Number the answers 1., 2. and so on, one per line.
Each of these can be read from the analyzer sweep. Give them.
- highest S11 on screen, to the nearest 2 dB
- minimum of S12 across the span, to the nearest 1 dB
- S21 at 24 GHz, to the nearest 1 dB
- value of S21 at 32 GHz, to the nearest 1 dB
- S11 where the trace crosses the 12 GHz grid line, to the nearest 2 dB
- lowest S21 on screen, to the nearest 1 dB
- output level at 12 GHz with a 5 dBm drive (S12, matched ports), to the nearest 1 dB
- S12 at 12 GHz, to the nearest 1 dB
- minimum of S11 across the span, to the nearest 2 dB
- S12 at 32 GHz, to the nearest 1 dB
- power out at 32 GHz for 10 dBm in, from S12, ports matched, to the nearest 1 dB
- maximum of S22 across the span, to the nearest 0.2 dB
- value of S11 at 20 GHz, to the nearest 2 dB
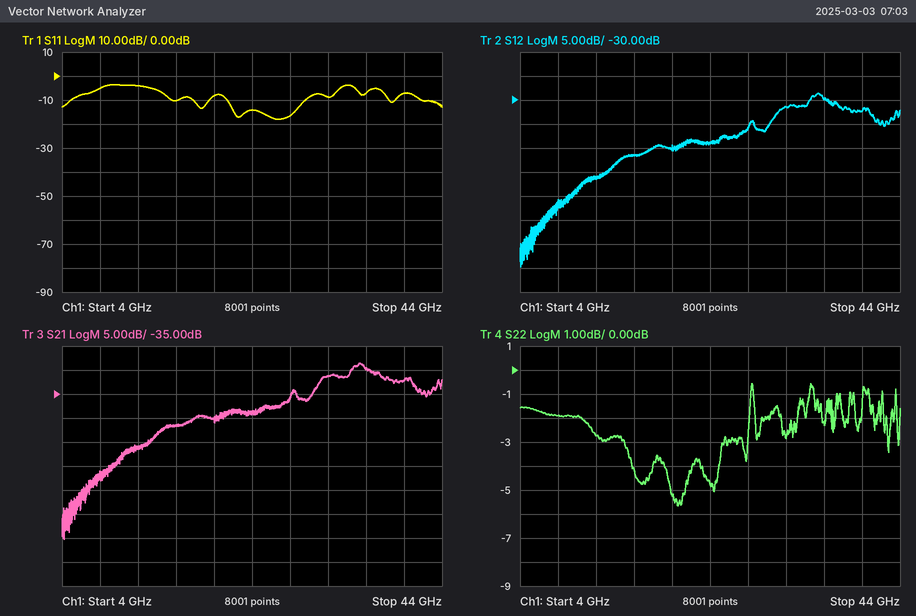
1. -4 dB
2. -65 dB
3. -39 dB
4. -31 dB
5. -4 dB
6. -65 dB
7. -41 dBm
8. -46 dB
9. -18 dB
10. -31 dB
11. -21 dBm
12. -0.6 dB
13. -8 dB
